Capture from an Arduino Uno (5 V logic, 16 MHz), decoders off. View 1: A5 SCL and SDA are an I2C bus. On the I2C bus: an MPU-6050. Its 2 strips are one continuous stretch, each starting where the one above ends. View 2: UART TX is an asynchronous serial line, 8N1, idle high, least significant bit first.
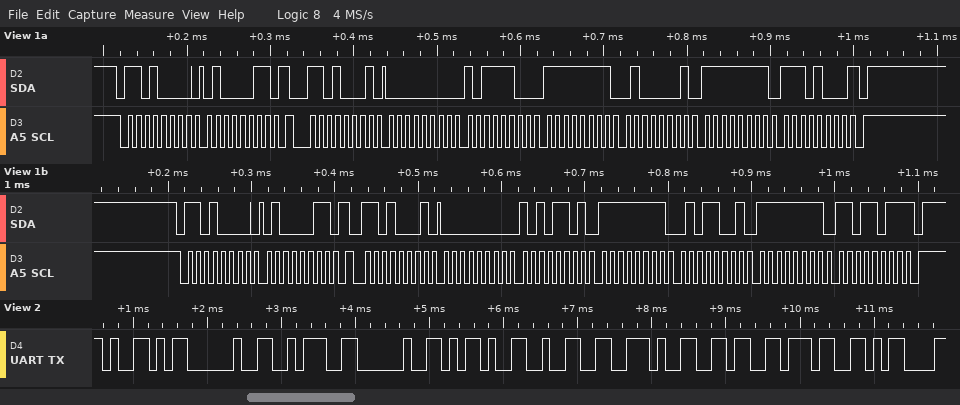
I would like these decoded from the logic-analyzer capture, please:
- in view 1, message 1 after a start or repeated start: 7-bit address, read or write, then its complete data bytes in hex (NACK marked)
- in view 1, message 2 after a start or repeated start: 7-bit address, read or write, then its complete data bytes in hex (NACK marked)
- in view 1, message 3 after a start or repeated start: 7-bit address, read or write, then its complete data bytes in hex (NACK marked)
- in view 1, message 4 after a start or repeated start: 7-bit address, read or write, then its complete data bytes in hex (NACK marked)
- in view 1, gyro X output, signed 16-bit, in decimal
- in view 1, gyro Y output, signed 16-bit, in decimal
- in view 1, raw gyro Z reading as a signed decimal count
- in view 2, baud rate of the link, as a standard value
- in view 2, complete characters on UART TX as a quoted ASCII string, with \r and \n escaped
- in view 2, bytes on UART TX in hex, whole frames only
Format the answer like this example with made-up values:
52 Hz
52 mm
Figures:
0x68 write: 43
0x68 read: 00 BC FF 41 FF E8 NACK
0x68 write: 43
0x68 read: 00 AD FF 59 FF DB NACK
188
-191
-24
9600 baud
"Y : -2.67\r"
59 20 3A 20 2D 32 2E 36 37 0D
